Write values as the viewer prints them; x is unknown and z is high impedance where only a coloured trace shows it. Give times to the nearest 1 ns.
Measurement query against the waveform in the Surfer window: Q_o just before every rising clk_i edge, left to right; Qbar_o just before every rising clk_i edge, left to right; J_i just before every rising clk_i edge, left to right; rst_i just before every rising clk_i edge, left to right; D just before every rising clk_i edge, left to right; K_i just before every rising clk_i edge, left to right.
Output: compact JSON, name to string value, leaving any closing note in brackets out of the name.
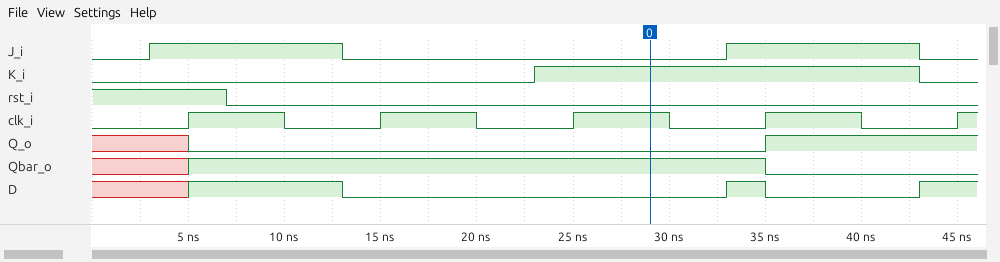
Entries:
{"Q_o just before every rising clk_i edge, left to right": "x 0 0 0 1", "Qbar_o just before every rising clk_i edge, left to right": "x 1 1 1 0", "J_i just before every rising clk_i edge, left to right": "1 0 0 1 0", "rst_i just before every rising clk_i edge, left to right": "1 0 0 0 0", "D just before every rising clk_i edge, left to right": "x 0 0 1 1", "K_i just before every rising clk_i edge, left to right": "0 0 1 1 0"}
